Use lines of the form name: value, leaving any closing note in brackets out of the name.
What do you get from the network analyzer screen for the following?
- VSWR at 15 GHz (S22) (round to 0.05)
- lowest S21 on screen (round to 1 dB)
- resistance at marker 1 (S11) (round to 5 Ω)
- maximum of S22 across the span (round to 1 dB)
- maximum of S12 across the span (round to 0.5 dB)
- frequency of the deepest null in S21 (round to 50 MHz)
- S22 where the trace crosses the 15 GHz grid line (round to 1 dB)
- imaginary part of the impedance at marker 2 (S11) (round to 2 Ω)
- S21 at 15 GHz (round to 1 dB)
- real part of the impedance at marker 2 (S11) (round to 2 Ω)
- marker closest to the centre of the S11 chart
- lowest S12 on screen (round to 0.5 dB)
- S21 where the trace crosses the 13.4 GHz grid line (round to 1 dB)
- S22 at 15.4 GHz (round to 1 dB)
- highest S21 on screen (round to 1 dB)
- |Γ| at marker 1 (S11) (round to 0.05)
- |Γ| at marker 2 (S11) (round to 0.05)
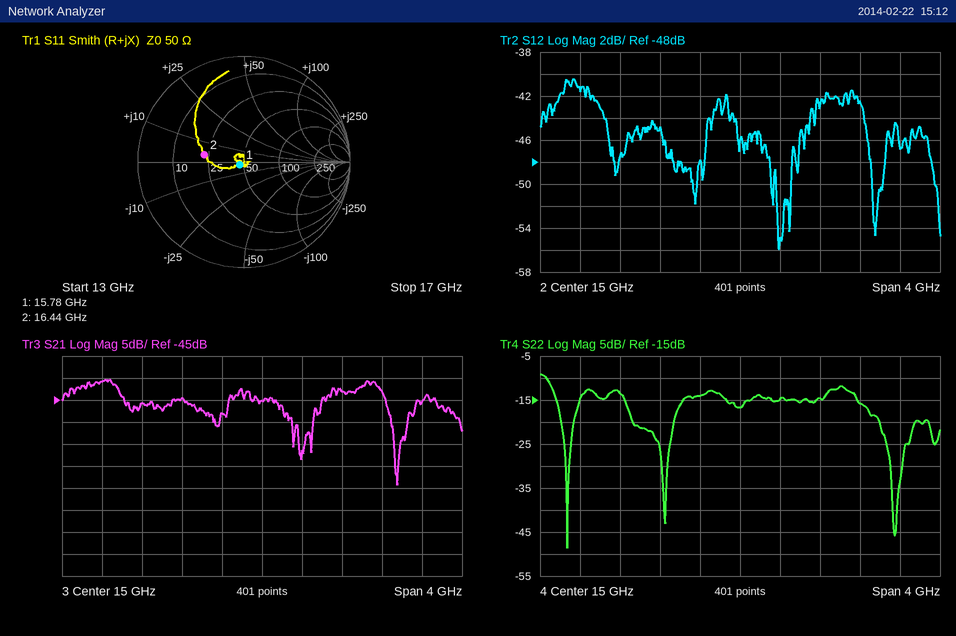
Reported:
VSWR at 15 GHz (S22): 1.35
lowest S21 on screen: -64 dB
resistance at marker 1 (S11): 45 Ω
maximum of S22 across the span: -9 dB
maximum of S12 across the span: -40.5 dB
frequency of the deepest null in S21: 16.35 GHz
S22 where the trace crosses the 15 GHz grid line: -17 dB
imaginary part of the impedance at marker 2 (S11): +4 Ω
S21 at 15 GHz: -45 dB
real part of the impedance at marker 2 (S11): 22 Ω
marker closest to the centre of the S11 chart: marker 1
lowest S12 on screen: -56.0 dB
S21 where the trace crosses the 13.4 GHz grid line: -41 dB
S22 at 15.4 GHz: -15 dB
highest S21 on screen: -40 dB
|Γ| at marker 1 (S11): 0.05
|Γ| at marker 2 (S11): 0.40
